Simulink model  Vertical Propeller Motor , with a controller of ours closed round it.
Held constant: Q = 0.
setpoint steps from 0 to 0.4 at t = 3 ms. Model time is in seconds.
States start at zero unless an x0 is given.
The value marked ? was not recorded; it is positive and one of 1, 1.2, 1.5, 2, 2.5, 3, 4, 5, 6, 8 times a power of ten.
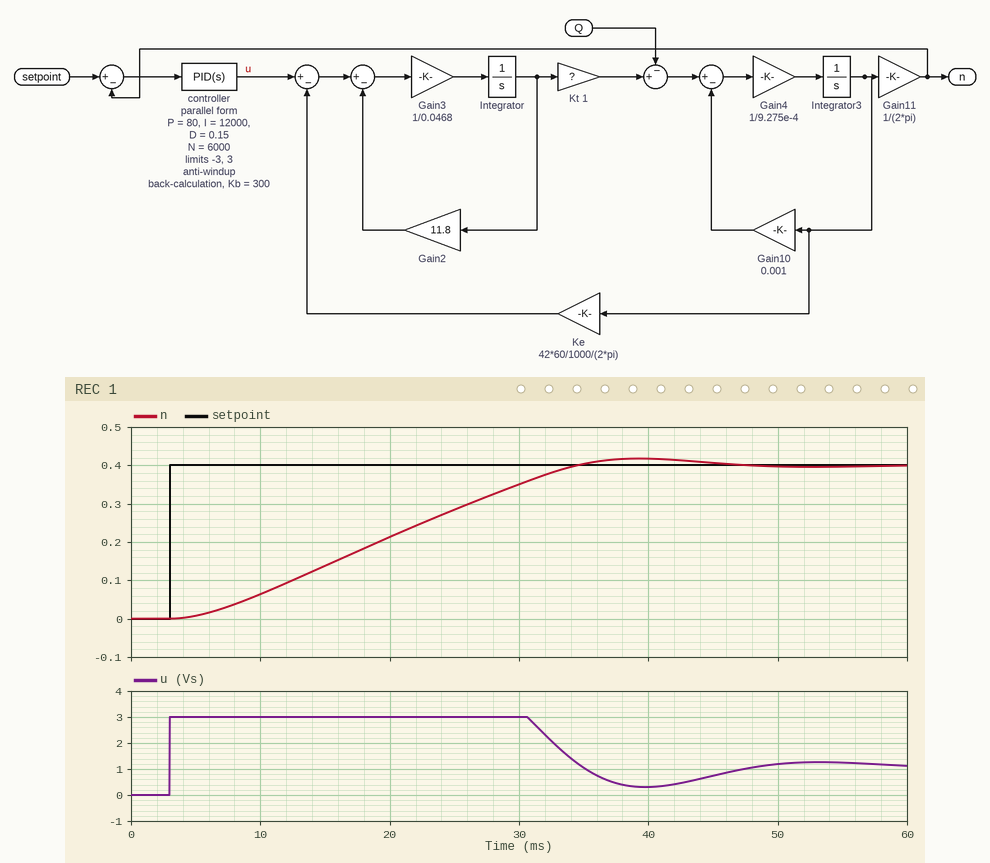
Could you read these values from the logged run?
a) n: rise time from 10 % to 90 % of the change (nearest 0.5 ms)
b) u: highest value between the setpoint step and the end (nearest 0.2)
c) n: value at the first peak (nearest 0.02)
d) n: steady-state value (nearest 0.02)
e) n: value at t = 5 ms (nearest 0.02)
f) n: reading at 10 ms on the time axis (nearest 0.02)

22.5 ms
3.0
0.42
0.40
0.00
0.06
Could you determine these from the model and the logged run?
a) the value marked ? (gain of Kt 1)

0.4
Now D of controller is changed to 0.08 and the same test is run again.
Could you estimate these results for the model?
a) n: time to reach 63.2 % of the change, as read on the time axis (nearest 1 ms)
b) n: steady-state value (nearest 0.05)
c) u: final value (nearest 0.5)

23 ms
0.40
1.0
